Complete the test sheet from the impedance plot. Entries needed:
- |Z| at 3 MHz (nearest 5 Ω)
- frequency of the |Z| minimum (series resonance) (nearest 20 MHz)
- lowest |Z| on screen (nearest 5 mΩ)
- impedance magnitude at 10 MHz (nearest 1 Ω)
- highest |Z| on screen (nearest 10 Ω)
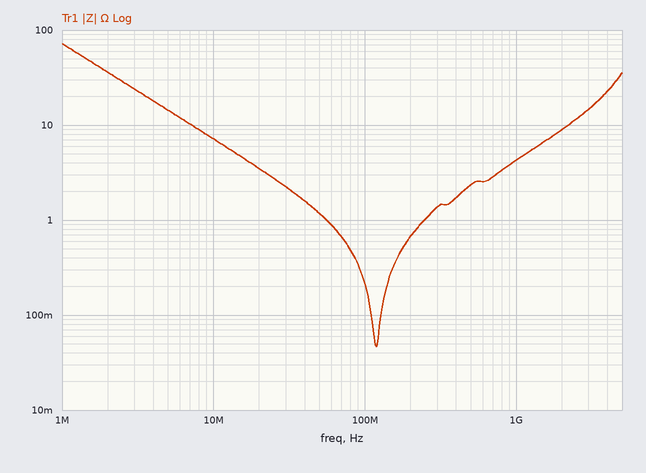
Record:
25 Ω
120 MHz
45 mΩ
7 Ω
70 Ω
